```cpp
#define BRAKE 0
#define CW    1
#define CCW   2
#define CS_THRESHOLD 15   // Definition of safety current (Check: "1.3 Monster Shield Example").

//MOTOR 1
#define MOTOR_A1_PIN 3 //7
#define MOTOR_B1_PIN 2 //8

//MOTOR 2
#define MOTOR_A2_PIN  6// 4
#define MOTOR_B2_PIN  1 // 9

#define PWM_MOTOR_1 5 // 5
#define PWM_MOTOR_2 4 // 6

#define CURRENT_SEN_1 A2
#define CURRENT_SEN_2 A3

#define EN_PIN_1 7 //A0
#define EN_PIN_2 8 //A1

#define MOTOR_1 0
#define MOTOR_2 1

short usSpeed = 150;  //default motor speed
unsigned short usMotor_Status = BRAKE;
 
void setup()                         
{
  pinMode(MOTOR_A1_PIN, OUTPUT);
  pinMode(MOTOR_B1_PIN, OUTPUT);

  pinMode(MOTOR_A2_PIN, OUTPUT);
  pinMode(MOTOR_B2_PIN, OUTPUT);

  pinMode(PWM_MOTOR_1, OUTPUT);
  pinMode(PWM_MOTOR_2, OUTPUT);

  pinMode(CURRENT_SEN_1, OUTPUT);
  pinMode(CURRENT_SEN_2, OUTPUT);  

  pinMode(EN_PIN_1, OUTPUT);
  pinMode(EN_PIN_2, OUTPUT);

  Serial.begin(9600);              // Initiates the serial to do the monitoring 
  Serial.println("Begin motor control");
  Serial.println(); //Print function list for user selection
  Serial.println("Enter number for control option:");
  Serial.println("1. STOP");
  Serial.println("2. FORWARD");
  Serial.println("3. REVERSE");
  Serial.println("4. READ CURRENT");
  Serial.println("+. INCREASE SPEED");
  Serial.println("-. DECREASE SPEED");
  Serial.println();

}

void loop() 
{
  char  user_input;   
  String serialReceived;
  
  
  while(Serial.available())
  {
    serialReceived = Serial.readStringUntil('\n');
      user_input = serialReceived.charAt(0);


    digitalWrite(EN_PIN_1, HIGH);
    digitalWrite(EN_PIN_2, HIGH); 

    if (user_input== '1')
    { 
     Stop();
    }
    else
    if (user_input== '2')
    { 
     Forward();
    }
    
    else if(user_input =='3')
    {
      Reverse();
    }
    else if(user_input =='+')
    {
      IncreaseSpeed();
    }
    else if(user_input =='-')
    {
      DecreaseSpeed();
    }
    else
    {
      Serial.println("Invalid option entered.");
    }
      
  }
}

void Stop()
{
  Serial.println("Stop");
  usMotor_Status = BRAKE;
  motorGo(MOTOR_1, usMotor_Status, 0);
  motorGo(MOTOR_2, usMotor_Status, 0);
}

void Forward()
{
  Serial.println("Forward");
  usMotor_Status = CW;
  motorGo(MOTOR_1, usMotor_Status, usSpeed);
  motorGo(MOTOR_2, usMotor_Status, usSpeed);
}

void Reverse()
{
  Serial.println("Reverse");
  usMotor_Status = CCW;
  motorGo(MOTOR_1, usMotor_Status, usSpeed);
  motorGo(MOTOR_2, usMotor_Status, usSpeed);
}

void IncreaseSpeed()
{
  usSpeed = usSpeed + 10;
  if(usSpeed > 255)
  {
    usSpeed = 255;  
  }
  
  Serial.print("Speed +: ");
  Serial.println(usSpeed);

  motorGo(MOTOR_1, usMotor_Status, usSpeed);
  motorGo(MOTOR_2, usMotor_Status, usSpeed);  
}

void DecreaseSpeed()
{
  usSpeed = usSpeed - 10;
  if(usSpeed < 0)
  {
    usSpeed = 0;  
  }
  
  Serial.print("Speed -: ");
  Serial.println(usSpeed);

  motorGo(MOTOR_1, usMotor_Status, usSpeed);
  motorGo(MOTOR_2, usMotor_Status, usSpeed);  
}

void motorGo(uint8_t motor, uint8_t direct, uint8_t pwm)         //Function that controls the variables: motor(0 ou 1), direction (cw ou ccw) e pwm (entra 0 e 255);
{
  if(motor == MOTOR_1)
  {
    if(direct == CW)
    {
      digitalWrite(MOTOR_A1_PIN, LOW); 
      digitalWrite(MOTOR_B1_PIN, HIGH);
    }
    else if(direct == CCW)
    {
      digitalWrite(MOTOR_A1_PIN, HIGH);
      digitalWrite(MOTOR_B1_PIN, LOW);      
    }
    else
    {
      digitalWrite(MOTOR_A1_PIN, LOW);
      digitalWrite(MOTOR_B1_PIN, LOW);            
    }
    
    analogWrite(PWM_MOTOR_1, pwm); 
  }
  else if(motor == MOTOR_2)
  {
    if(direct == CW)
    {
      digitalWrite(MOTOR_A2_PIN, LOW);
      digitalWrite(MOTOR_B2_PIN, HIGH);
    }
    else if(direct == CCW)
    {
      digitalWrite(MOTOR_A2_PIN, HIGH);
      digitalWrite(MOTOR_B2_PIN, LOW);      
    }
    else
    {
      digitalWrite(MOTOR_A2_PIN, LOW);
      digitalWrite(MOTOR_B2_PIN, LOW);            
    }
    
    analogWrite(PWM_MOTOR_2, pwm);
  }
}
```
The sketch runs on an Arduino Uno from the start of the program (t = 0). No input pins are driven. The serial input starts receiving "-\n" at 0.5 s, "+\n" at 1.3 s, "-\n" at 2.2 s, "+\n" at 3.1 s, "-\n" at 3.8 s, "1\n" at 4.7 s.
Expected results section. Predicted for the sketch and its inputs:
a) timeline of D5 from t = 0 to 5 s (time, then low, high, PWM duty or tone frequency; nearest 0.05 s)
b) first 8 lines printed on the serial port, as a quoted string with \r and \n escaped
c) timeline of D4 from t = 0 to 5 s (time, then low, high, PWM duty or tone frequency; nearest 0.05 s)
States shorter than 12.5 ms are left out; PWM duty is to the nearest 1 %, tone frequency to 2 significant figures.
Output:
0 s low; 0.5 s PWM 55 %; 1.3 s PWM 59 %; 2.2 s PWM 55 %; 3.1 s PWM 59 %; 3.8 s PWM 55 %; 4.7 s low
"Begin motor control\r\n\r\nEnter number for control option:\r\n1. STOP\r\n2. FORWARD\r\n3. REVERSE\r\n4. READ CURRENT\r\n+. INCREASE SPEED\r\n"
0 s low; 0.5 s high; 4.7 s low
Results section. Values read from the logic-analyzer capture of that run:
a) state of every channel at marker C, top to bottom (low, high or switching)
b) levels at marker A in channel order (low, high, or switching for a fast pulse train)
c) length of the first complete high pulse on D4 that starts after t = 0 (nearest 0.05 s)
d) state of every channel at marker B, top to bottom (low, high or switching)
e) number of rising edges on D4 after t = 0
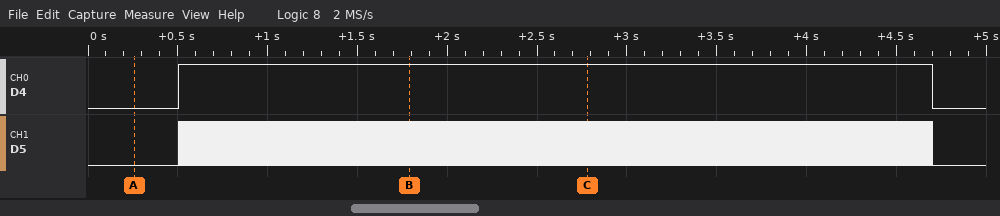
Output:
D4 high, D5 switching
D4 low, D5 low
4.20 s
D4 high, D5 switching
1
